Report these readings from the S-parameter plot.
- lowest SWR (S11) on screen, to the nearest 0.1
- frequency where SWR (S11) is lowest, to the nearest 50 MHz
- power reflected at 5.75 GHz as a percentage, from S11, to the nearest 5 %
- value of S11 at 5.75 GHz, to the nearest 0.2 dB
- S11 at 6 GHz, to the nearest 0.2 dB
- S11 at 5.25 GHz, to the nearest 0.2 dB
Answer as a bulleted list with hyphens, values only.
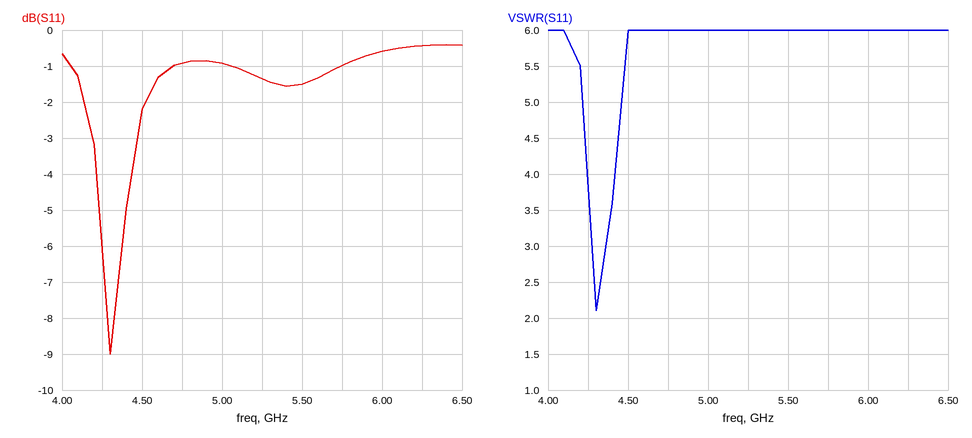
- 2.1
- 4.30 GHz
- 80 %
- -1.0 dB
- -0.6 dB
- -1.4 dB
